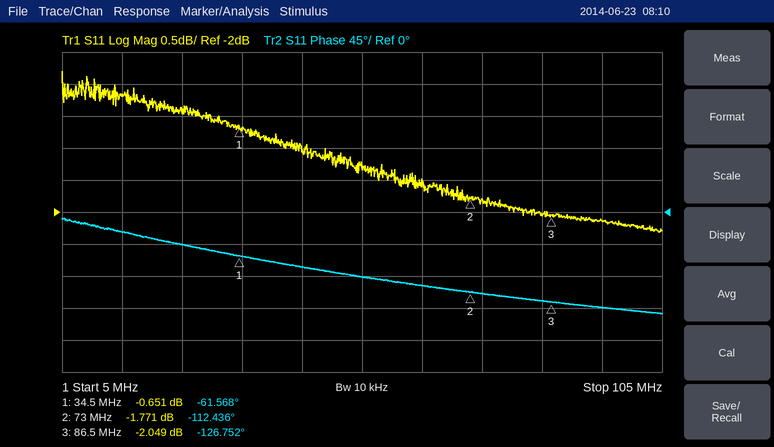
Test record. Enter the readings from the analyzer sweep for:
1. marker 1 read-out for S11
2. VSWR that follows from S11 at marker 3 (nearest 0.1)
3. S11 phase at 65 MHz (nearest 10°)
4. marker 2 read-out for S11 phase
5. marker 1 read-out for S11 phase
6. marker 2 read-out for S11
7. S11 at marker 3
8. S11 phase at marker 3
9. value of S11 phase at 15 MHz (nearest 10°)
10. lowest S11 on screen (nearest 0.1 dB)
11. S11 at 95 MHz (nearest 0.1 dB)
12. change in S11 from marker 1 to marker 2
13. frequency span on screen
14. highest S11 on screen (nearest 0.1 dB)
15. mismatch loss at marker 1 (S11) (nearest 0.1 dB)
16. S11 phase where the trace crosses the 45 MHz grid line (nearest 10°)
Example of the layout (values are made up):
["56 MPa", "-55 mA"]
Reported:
["-0.651 dB", "8.5", "-100°", "-112.436°", "-61.568°", "-1.771 dB", "-2.049 dB", "-126.752°", "-30°", "-2.3 dB", "-2.1 dB", "-1.120 dB", "100 MHz", "0.2 dB", "8.6 dB", "-80°"]
